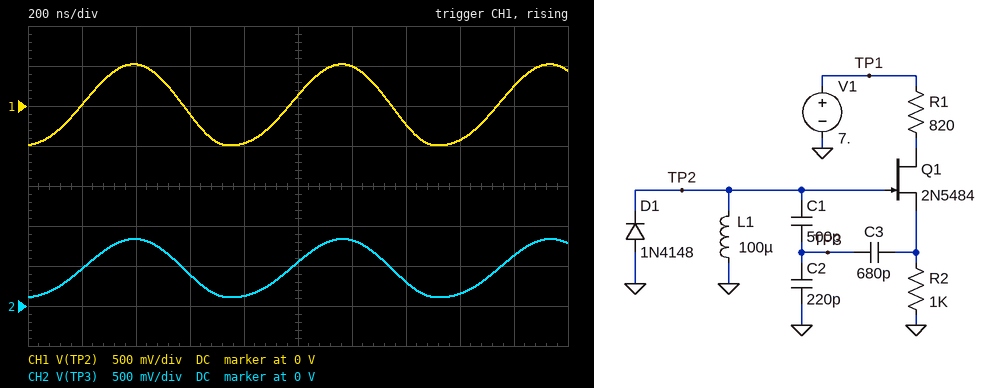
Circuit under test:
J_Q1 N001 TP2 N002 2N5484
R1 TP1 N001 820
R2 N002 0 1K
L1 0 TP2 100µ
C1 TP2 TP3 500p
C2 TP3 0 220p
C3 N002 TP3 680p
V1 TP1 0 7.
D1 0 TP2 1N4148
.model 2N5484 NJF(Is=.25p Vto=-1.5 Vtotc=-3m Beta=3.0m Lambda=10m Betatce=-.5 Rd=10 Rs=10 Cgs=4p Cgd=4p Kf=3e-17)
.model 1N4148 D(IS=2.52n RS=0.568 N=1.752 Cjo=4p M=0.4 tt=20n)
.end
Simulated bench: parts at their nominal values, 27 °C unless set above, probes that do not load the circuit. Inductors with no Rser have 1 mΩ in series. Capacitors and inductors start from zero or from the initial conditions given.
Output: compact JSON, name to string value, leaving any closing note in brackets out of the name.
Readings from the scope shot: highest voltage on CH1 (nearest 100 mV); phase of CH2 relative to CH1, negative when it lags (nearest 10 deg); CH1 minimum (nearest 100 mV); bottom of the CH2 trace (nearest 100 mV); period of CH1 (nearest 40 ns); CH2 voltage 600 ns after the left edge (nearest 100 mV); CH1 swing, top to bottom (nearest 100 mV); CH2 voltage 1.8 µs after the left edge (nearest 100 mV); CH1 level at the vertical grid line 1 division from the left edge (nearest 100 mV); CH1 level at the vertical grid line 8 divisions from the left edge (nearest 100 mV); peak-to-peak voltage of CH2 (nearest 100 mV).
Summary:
{"highest voltage on CH1": "500 mV", "phase of CH2 relative to CH1, negative when it lags": "0 deg", "CH1 minimum": "-500 mV", "bottom of the CH2 trace": "100 mV", "period of CH1": "760 ns", "CH2 voltage 600 ns after the left edge": "400 mV", "CH1 swing, top to bottom": "1.0 V", "CH2 voltage 1.8 µs after the left edge": "600 mV", "CH1 level at the vertical grid line 1 division from the left edge": "0 V", "CH1 level at the vertical grid line 8 divisions from the left edge": "-400 mV", "peak-to-peak voltage of CH2": "700 mV"}
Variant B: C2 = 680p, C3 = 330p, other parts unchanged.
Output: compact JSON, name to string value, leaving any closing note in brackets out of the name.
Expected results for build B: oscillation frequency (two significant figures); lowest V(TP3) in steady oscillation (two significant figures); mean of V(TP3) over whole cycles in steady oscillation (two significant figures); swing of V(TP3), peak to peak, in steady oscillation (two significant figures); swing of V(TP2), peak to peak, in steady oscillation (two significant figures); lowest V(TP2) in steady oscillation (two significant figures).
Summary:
{"oscillation frequency": "980 kHz", "lowest V(TP3) in steady oscillation": "-36 mV", "mean of V(TP3) over whole cycles in steady oscillation": "210 mV", "swing of V(TP3), peak to peak, in steady oscillation": "500 mV", "swing of V(TP2), peak to peak, in steady oscillation": "1.0 V", "lowest V(TP2) in steady oscillation": "-500 mV"}
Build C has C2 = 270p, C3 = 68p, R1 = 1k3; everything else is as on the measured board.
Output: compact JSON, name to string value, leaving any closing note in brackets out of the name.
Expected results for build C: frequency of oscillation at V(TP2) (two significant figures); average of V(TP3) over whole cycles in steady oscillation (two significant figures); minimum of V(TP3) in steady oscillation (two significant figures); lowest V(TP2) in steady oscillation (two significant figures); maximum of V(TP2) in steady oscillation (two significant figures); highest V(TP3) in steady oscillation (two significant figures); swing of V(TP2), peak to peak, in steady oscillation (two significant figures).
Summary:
{"frequency of oscillation at V(TP2)": "1.2 MHz", "average of V(TP3) over whole cycles in steady oscillation": "77 mV", "minimum of V(TP3) in steady oscillation": "-150 mV", "lowest V(TP2) in steady oscillation": "-340 mV", "maximum of V(TP2) in steady oscillation": "340 mV", "highest V(TP3) in steady oscillation": "300 mV", "swing of V(TP2), peak to peak, in steady oscillation": "680 mV"}
